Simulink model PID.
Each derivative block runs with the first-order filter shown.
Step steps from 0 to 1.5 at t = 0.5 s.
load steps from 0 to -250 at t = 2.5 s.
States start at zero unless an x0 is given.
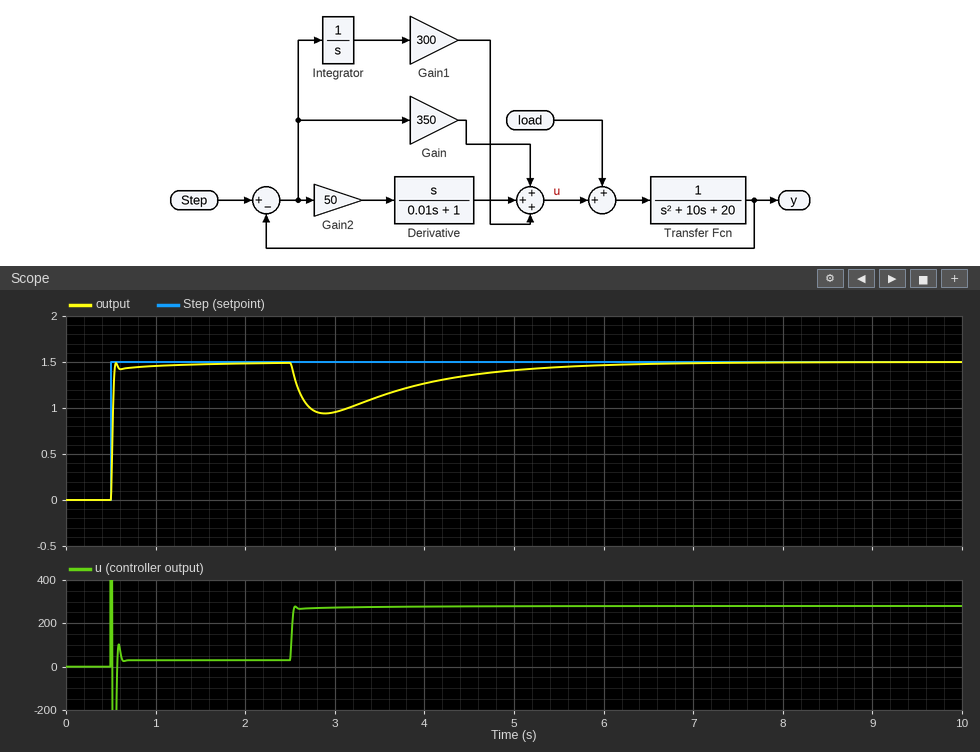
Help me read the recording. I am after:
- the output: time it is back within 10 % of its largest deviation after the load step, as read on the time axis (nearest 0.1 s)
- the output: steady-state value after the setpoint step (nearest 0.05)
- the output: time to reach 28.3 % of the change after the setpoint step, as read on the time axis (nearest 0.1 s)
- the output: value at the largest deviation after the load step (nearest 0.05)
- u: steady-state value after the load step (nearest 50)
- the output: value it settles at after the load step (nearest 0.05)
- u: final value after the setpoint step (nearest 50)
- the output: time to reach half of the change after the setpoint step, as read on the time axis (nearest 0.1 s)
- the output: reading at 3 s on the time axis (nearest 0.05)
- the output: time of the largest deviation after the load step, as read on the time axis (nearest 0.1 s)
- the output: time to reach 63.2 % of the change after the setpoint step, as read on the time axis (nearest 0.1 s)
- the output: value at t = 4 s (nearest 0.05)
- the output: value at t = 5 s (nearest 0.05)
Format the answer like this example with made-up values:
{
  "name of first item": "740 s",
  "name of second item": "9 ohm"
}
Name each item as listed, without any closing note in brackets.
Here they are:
{
  "the output: time it is back within 10 % of its largest deviation after the load step, as read on the time axis": "5.5 s",
  "the output: steady-state value after the setpoint step": "1.50",
  "the output: time to reach 28.3 % of the change after the setpoint step, as read on the time axis": "0.5 s",
  "the output: value at the largest deviation after the load step": "0.95",
  "u: steady-state value after the load step": "300",
  "the output: value it settles at after the load step": "1.50",
  "u: final value after the setpoint step": "50",
  "the output: time to reach half of the change after the setpoint step, as read on the time axis": "0.5 s",
  "the output: reading at 3 s on the time axis": "0.95",
  "the output: time of the largest deviation after the load step, as read on the time axis": "2.9 s",
  "the output: time to reach 63.2 % of the change after the setpoint step, as read on the time axis": "0.5 s",
  "the output: value at t = 4 s": "1.25",
  "the output: value at t = 5 s": "1.40"
}
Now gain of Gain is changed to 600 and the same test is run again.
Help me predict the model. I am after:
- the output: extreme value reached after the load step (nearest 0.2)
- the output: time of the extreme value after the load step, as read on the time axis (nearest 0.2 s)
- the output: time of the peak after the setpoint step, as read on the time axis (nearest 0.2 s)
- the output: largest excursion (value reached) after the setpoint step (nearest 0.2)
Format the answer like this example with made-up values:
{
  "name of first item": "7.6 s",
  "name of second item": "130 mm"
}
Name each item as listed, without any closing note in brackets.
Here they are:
{
  "the output: extreme value reached after the load step": "1.2",
  "the output: time of the extreme value after the load step, as read on the time axis": "2.8 s",
  "the output: time of the peak after the setpoint step, as read on the time axis": "0.6 s",
  "the output: largest excursion (value reached) after the setpoint step": "1.6"
}
